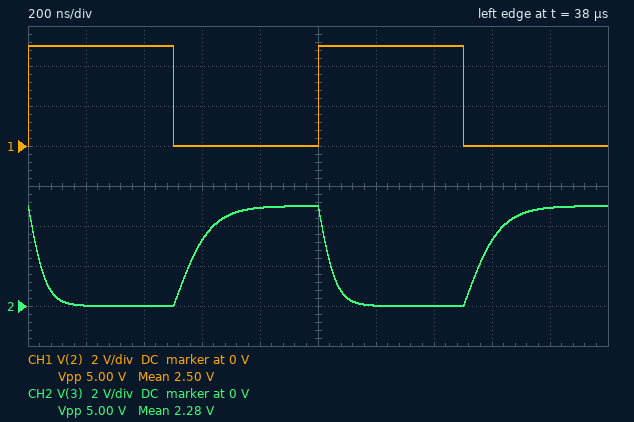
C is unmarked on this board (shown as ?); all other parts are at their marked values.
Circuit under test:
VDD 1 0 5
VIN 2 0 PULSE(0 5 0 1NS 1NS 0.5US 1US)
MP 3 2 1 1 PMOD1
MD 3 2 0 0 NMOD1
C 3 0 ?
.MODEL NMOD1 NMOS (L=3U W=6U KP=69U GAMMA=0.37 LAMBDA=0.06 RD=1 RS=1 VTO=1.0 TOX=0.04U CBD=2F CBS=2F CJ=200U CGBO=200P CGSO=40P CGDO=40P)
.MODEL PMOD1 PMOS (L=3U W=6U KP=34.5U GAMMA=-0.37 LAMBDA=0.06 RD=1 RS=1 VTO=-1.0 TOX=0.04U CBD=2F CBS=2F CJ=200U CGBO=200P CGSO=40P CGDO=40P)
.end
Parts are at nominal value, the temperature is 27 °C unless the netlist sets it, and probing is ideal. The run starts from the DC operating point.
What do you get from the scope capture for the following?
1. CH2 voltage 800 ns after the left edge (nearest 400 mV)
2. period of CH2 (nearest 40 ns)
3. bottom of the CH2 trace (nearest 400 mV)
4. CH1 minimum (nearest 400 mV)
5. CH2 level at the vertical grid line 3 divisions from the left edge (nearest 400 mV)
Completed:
4.8 V
1.00 µs
0 V
0 V
3.2 V
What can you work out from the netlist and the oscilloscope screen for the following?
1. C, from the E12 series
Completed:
18 pF
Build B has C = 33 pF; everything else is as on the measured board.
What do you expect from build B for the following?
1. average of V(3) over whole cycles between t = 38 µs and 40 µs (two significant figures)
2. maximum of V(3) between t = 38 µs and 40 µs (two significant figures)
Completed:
2.1 V
4.9 V
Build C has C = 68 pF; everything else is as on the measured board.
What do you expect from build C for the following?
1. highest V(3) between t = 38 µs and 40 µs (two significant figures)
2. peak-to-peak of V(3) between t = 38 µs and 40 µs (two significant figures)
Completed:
4.0 V
3.9 V
